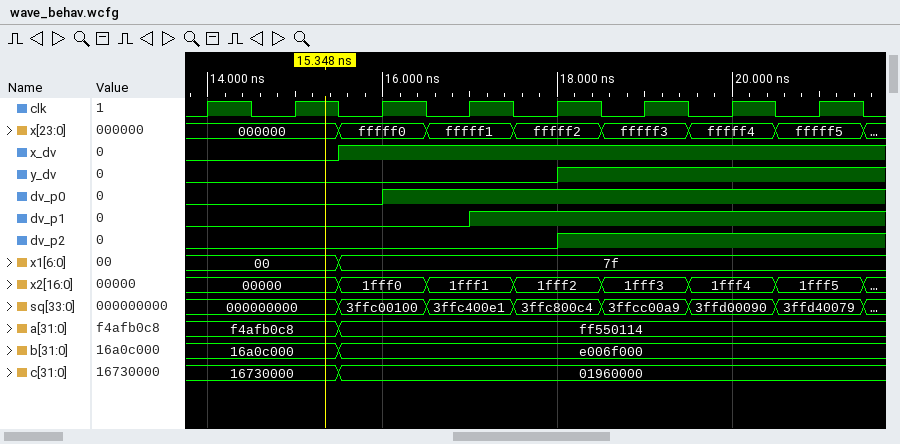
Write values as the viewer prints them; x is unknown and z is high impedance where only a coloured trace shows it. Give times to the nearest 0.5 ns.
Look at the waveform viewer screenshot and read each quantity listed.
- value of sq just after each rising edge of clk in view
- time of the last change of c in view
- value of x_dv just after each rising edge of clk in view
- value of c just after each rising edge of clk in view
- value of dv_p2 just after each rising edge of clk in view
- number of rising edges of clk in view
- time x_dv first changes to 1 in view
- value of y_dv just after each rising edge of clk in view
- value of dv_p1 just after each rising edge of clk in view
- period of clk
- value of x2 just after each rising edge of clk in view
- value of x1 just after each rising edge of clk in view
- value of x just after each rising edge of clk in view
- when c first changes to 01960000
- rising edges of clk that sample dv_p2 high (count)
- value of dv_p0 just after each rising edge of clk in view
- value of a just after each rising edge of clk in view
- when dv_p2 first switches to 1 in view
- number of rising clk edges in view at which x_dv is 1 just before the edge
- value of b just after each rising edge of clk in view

000000000, 000000000, 3ffc00100, 3ffc400e1, 3ffc800c4, 3ffcc00a9, 3ffd00090, 3ffd40079
15.5 ns
0 0 1 1 1 1 1 1
16730000, 16730000, 01960000, 01960000, 01960000, 01960000, 01960000, 01960000
0 0 0 0 1 1 1 1
8
15.5 ns
0 0 0 0 1 1 1 1
0 0 0 1 1 1 1 1
1 ns
00000, 00000, 1fff0, 1fff1, 1fff2, 1fff3, 1fff4, 1fff5
00, 00, 7f, 7f, 7f, 7f, 7f, 7f
000000, 000000, fffff0, fffff1, fffff2, fffff3, fffff4, fffff5
15.5 ns
3
0 0 1 1 1 1 1 1
f4afb0c8, f4afb0c8, ff550114, ff550114, ff550114, ff550114, ff550114, ff550114
18 ns
6
16a0c000, 16a0c000, e006f000, e006f000, e006f000, e006f000, e006f000, e006f000
